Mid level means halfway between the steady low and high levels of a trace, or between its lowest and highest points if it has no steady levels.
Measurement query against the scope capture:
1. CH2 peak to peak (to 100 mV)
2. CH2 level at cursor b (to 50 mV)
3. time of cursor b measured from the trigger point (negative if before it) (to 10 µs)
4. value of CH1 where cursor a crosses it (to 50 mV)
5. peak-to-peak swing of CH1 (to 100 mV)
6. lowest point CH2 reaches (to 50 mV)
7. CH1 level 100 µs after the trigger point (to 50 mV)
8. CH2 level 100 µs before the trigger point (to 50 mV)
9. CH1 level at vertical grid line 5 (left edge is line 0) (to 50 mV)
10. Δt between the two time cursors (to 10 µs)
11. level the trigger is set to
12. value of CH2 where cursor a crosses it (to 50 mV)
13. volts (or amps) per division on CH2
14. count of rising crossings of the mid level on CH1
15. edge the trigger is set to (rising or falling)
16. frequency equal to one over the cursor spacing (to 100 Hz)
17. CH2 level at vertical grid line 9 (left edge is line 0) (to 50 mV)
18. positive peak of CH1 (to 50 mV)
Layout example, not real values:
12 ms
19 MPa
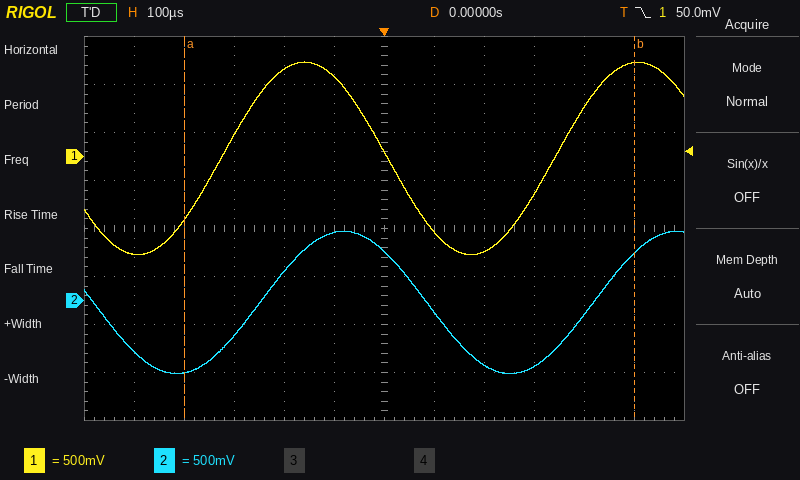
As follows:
1.50 V
500 mV
+500 µs
-650 mV
2.00 V
-750 mV
-800 mV
700 mV
850 mV
900 µs
50.0 mV
-750 mV
500 mV
2
falling
1.1 kHz
-700 mV
1.00 V
